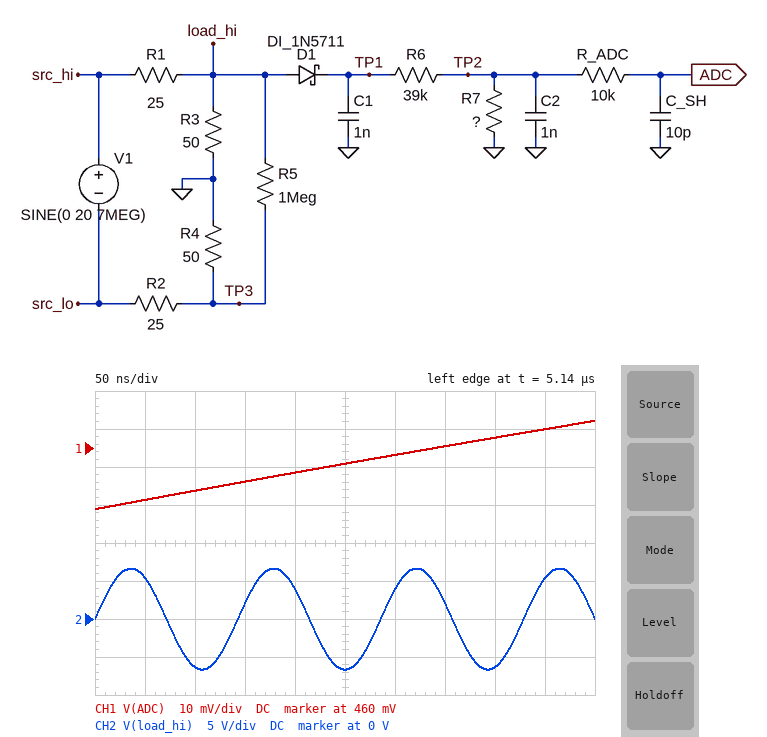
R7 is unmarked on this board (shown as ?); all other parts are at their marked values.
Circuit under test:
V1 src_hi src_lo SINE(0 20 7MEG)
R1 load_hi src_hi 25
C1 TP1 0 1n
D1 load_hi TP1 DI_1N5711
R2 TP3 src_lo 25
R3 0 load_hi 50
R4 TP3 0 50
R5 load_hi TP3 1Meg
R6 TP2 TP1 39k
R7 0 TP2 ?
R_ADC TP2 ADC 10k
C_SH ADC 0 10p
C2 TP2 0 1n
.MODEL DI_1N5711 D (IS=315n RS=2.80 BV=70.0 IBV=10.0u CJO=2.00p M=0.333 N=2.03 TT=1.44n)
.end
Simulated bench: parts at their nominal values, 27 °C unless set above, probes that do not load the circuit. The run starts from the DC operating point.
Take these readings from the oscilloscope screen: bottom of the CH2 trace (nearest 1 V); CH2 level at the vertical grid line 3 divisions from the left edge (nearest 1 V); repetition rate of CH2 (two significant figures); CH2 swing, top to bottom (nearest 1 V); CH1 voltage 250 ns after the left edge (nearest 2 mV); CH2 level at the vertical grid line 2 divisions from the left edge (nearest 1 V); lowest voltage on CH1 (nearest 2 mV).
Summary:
-7 V
2 V
7.0 MHz
13 V
456 mV
-6 V
444 mV
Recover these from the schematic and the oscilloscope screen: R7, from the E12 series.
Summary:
4.7 kΩ
